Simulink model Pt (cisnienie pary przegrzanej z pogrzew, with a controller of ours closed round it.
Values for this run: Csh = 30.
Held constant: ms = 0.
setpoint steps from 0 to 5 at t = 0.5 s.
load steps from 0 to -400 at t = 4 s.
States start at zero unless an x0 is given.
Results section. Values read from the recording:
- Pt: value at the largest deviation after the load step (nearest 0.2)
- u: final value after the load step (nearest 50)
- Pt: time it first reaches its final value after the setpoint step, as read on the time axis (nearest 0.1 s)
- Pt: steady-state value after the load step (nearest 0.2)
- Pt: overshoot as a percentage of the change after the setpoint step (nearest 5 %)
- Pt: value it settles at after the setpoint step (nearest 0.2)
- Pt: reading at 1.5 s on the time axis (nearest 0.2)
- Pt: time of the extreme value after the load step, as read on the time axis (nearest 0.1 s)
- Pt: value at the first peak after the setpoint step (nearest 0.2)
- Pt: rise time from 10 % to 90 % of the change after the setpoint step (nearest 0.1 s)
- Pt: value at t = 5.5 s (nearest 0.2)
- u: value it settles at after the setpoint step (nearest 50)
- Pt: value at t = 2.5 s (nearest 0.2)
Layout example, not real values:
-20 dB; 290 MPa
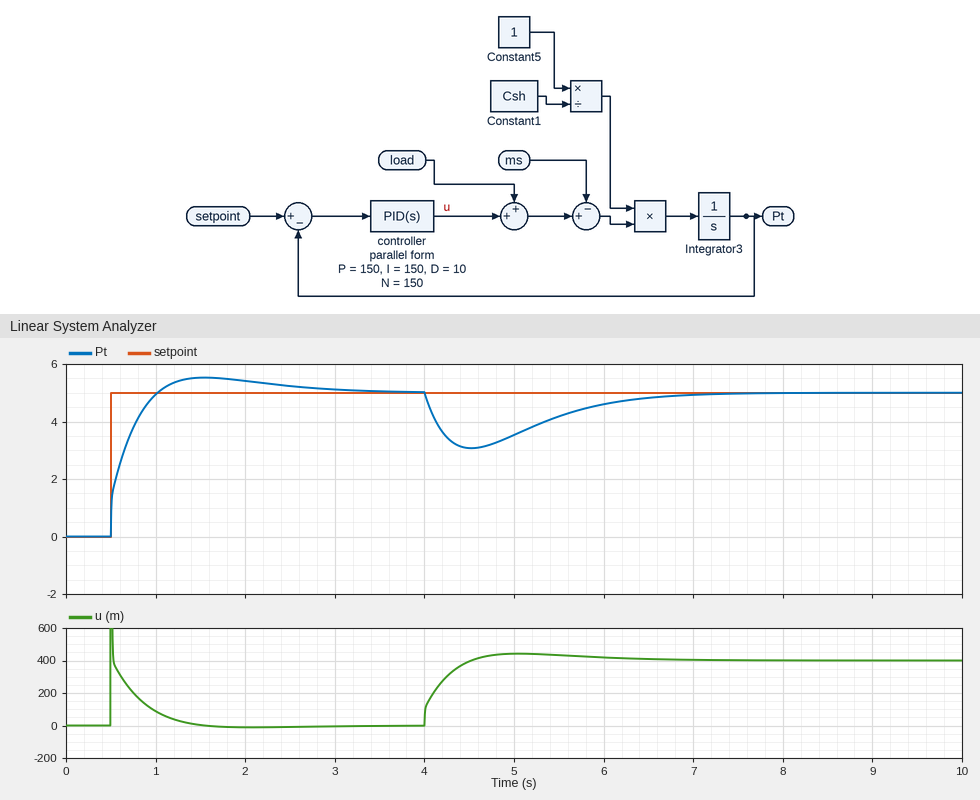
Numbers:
3.0; 400; 1.0 s; 5.0; 10 %; 5.0; 5.6; 4.5 s; 5.6; 0.4 s; 4.2; 0; 5.2
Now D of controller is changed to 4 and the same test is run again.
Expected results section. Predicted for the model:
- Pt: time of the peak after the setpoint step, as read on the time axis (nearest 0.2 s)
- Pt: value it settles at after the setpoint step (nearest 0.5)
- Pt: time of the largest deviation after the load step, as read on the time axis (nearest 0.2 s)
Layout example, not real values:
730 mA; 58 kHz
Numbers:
1.4 s; 5.0; 4.4 s
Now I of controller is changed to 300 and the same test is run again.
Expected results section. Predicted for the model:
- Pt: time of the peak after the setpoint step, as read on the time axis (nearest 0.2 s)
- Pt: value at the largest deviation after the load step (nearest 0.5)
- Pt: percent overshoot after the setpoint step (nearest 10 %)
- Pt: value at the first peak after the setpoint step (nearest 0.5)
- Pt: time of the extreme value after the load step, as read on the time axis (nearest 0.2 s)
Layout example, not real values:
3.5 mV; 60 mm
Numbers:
1.4 s; 3.5; 20 %; 6.0; 4.4 s
